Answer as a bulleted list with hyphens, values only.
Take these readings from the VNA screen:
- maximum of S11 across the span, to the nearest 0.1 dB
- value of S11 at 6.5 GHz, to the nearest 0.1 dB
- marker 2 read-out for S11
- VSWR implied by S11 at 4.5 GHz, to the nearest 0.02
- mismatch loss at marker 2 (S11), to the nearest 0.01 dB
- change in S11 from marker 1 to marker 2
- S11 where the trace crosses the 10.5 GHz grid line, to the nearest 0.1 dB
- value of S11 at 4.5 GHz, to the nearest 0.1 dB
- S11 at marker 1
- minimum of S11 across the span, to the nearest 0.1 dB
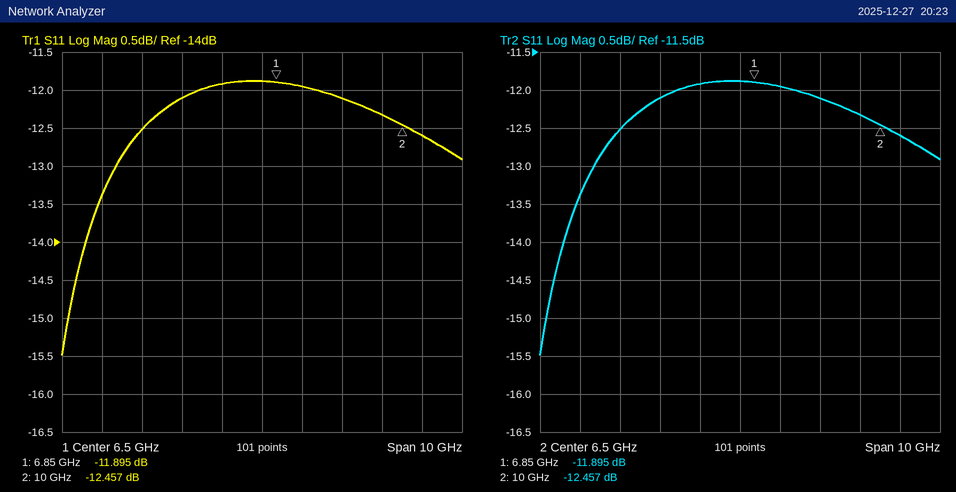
- -11.9 dB
- -11.9 dB
- -12.457 dB
- 1.66
- 0.25 dB
- -0.562 dB
- -12.6 dB
- -12.1 dB
- -11.895 dB
- -15.5 dB
